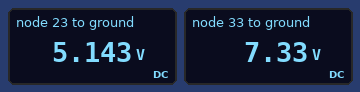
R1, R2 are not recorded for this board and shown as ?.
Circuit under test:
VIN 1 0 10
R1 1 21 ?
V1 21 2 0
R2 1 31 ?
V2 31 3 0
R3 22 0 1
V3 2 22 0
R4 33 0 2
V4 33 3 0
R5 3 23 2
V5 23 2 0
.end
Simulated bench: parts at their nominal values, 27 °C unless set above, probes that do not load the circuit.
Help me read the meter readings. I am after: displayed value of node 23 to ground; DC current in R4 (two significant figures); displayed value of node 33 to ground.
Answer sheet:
5.143 V
3.7 A
7.33 V
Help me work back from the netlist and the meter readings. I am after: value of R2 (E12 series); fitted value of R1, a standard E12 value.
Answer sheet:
0.56 Ω
1.2 Ω
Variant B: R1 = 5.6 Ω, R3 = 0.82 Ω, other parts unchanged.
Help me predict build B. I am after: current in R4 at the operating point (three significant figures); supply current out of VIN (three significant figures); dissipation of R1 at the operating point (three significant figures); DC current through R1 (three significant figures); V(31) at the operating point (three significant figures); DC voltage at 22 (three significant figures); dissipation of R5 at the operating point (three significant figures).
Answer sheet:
3.45 A
6.82 A
9.36 W
1.29 A
6.91 V
2.76 V
8.59 W
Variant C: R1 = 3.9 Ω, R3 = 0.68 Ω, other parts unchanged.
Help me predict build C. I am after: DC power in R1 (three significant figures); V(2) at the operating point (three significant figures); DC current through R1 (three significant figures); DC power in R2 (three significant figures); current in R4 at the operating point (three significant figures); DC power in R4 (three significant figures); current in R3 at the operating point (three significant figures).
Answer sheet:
13.7 W
2.70 V
1.87 A
17.2 W
3.45 A
23.8 W
3.97 A
